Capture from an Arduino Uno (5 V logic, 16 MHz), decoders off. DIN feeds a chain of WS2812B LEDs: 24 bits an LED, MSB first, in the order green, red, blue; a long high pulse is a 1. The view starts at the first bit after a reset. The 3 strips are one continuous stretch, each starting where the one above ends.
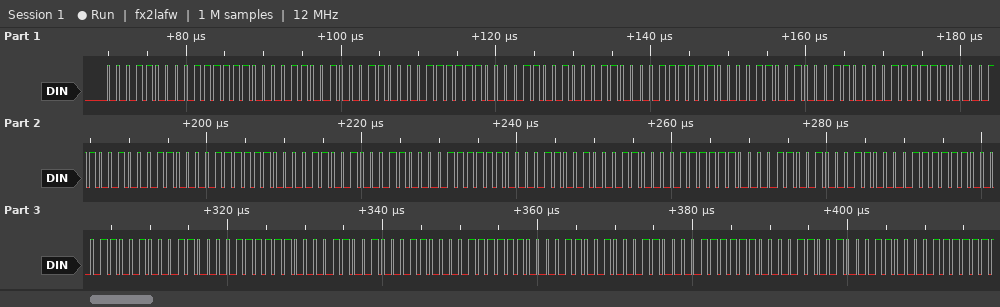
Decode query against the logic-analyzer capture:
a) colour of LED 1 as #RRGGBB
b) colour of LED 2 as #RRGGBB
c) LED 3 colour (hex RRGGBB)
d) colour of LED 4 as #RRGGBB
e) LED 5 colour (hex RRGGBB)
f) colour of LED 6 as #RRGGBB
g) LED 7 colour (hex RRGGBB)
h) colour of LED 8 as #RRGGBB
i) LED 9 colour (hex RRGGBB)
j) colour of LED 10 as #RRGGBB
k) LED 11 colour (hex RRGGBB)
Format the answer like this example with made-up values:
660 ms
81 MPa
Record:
#7E1819
#7E1819
#7E1819
#7E1819
#7E1819
#7E1819
#7E1819
#7E1819
#7E1819
#7E1819
#7E1819
